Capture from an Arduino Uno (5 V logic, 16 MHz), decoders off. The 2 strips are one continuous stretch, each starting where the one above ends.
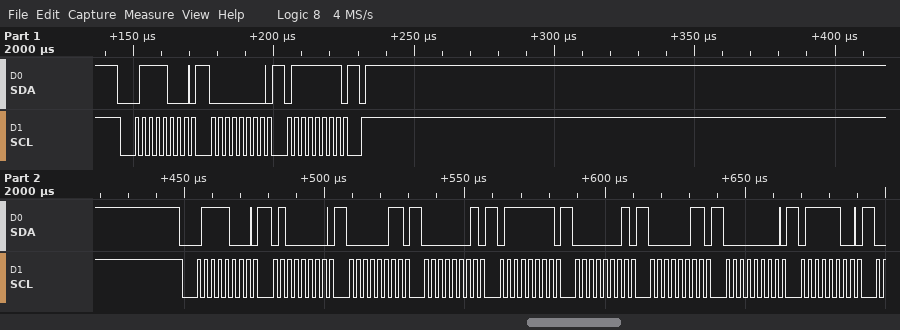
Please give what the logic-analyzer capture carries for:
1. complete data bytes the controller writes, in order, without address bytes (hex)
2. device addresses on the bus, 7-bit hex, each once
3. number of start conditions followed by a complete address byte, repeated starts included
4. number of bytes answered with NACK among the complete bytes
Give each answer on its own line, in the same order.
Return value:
00 7F 40 03 01 7F 01 03 00 7C
0x3C
2
0
